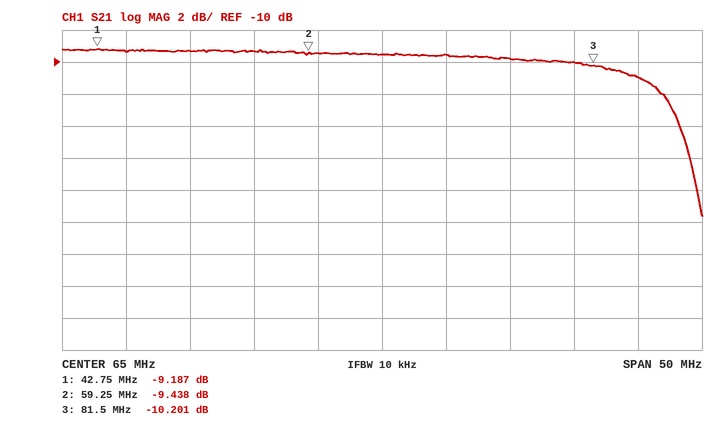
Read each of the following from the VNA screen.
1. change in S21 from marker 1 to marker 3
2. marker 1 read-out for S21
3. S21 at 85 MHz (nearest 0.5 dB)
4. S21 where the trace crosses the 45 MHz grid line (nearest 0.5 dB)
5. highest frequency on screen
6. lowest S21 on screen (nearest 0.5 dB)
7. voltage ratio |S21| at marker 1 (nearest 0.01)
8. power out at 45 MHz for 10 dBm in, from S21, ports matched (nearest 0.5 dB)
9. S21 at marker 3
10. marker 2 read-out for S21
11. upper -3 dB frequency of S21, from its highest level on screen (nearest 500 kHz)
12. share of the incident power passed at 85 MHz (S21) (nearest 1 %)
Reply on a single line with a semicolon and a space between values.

-1.014 dB; -9.187 dB; -11.0 dB; -9.5 dB; 90 MHz; -19.5 dB; 0.35; 0.5 dBm; -10.201 dB; -9.438 dB; 87.0 MHz; 8 %
